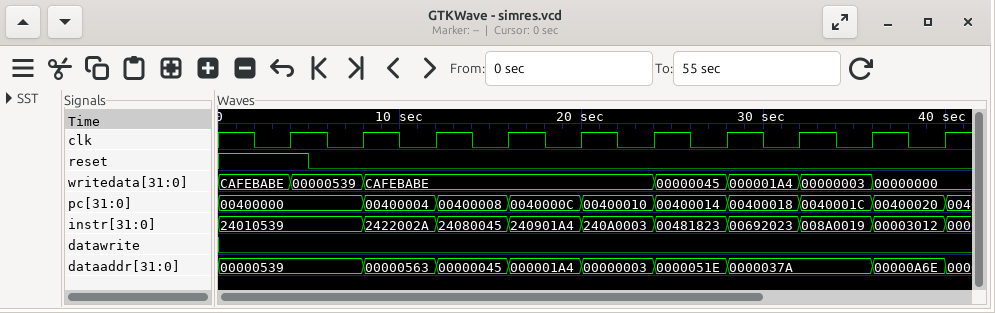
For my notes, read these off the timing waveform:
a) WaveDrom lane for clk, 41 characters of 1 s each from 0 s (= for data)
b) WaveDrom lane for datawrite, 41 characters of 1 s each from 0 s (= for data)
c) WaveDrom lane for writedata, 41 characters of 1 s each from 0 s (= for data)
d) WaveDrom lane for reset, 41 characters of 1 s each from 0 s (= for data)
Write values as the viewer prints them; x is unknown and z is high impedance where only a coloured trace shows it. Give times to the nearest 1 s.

{name: 'clk', wave: '1.0.1.0.1.0.1.0.1.0.1.0.1.0.1.0.1.0.1.0.1'}
{name: 'datawrite', wave: '0........................................'}
{name: 'writedata', wave: '=...=...=...............=...=...=...=....', data: 'CAFEBABE 00000539 CAFEBABE 00000045 000001A4 00000003 00000000'}
{name: 'reset', wave: '1....0...................................'}
